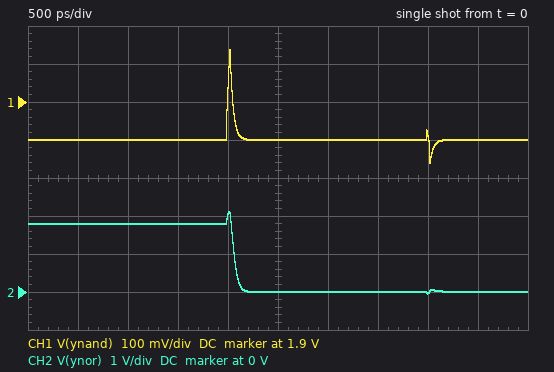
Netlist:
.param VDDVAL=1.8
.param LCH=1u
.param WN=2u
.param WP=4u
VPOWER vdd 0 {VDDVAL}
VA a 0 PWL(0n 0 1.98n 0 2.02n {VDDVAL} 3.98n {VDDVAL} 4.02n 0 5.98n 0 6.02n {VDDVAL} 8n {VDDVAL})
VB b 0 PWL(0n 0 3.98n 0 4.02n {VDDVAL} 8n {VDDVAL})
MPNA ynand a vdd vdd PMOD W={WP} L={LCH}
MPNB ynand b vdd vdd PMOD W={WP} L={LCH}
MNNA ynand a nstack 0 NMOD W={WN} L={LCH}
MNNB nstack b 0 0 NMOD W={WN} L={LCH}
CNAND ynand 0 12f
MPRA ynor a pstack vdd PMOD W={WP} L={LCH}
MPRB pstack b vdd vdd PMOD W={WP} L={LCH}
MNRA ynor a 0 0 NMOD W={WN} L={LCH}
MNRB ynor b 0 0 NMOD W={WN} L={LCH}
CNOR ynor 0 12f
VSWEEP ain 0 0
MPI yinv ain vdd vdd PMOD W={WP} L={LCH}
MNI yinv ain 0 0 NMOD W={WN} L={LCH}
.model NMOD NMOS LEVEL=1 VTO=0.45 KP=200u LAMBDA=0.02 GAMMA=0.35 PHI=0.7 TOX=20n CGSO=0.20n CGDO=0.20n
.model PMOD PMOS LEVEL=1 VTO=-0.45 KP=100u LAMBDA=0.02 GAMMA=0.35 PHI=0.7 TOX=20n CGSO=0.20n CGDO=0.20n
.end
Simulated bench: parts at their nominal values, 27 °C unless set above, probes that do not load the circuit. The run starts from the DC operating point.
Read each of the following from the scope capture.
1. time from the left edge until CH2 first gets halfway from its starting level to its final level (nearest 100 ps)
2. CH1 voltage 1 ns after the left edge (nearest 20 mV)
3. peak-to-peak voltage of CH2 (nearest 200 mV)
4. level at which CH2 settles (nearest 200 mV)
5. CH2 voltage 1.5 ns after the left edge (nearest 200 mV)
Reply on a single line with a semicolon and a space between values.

2.1 ns; 1.80 V; 2.2 V; 0 V; 1.8 V
